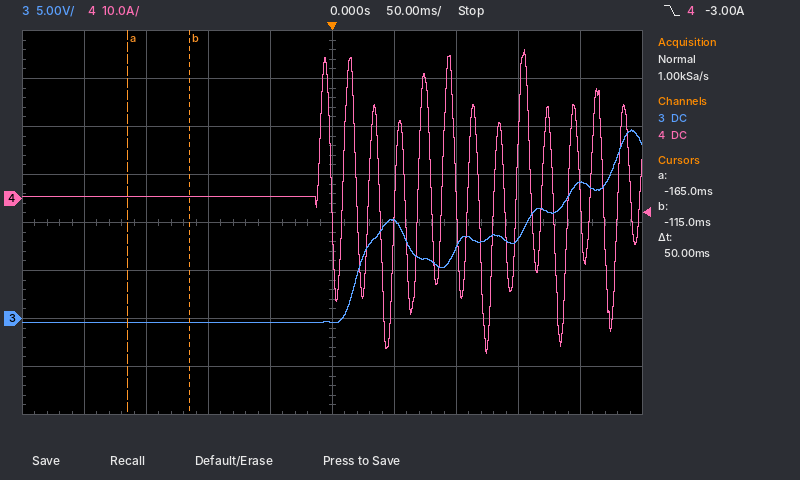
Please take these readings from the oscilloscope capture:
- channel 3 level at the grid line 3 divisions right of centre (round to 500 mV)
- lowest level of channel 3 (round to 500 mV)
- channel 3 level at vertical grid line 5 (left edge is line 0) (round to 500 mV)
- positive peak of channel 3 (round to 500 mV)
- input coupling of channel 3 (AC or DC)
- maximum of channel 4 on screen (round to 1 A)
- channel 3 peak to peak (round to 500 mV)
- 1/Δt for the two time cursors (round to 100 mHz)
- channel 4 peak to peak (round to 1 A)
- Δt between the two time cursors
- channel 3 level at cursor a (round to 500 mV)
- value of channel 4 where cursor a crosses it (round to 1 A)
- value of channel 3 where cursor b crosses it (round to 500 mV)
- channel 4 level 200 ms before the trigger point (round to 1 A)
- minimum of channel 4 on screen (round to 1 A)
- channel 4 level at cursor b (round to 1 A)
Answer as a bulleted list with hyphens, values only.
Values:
- 8.5 V
- -500 mV
- -500 mV
- 19.5 V
- DC
- 31 A
- 20.0 V
- 20.0 Hz
- 63 A
- 50 ms
- -500 mV
- 0 A
- -500 mV
- 0 A
- -32 A
- 0 A
